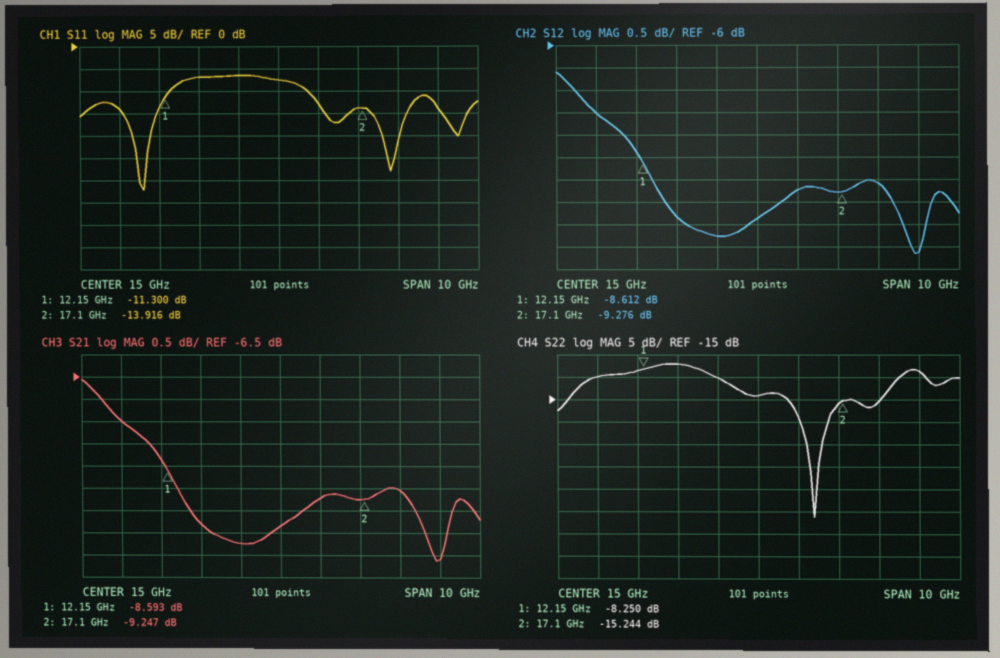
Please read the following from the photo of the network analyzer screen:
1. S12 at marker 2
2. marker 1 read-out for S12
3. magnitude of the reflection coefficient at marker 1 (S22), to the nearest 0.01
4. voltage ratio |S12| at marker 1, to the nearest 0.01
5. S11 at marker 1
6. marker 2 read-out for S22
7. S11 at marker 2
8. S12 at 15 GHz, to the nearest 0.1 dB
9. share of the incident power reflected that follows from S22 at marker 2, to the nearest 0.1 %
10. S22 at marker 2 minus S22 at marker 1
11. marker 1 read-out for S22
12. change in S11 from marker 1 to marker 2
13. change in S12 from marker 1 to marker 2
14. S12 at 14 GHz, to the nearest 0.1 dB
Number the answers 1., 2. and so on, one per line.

1. -9.276 dB
2. -8.612 dB
3. 0.39
4. 0.37
5. -11.300 dB
6. -15.244 dB
7. -13.916 dB
8. -9.9 dB
9. 3.0 %
10. -6.994 dB
11. -8.250 dB
12. -2.616 dB
13. -0.664 dB
14. -10.3 dB
